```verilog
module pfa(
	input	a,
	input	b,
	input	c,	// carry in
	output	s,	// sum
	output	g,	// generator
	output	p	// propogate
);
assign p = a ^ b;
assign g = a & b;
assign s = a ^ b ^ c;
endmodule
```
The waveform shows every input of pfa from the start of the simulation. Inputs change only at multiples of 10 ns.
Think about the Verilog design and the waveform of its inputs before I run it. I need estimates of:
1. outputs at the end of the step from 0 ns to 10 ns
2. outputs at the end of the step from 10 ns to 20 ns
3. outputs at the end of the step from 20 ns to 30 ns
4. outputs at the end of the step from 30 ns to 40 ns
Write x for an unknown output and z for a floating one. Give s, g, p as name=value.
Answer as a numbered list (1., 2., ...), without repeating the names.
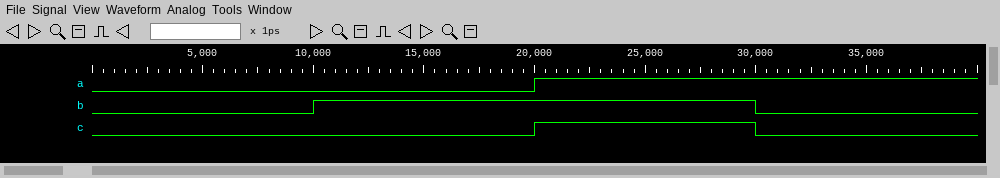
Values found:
1. s=0, g=0, p=0
2. s=1, g=0, p=1
3. s=1, g=1, p=0
4. s=1, g=0, p=1
